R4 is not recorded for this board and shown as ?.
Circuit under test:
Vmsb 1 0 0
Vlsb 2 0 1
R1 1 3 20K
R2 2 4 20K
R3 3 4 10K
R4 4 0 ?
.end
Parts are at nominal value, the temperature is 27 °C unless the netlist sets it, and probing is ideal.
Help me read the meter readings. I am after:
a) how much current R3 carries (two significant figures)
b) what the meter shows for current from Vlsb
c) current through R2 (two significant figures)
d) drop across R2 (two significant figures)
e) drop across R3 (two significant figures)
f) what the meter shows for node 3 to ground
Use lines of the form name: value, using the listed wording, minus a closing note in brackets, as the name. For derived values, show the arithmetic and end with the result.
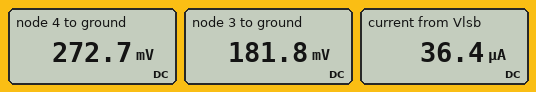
how much current R3 carries: (272.7 mV - 181.8 mV) / 10 kΩ = 9.1 µA
what the meter shows for current from Vlsb: 36.4 µA
current through R2: (1 V - 272.7 mV) / 20 kΩ = 36 µA
drop across R2: 1 V - 272.7 mV = 730 mV
drop across R3: 272.7 mV - 181.8 mV = 91 mV
what the meter shows for node 3 to ground: 181.8 mV
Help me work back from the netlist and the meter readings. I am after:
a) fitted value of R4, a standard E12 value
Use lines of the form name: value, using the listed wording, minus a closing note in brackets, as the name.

fitted value of R4, a standard E12 value: 10 kΩ
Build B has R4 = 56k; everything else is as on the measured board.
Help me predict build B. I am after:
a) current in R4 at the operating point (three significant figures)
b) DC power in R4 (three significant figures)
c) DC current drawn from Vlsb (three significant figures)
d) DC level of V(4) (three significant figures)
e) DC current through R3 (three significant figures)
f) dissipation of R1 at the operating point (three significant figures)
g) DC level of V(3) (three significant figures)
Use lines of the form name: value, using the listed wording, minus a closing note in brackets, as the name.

current in R4 at the operating point: 8.82 µA
DC power in R4: 4.36 µW
DC current drawn from Vlsb: 25.3 µA
DC level of V(4): 494 mV
DC current through R3: 16.5 µA
dissipation of R1 at the operating point: 5.43 µW
DC level of V(3): 329 mV
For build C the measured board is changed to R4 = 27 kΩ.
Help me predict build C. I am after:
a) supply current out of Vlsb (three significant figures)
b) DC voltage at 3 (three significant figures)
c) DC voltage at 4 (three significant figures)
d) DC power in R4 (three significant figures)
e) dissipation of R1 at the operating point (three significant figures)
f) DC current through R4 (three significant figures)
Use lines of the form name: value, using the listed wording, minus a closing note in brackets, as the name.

supply current out of Vlsb: 29.2 µA
DC voltage at 3: 277 mV
DC voltage at 4: 415 mV
DC power in R4: 6.39 µW
dissipation of R1 at the operating point: 3.83 µW
DC current through R4: 15.4 µA
